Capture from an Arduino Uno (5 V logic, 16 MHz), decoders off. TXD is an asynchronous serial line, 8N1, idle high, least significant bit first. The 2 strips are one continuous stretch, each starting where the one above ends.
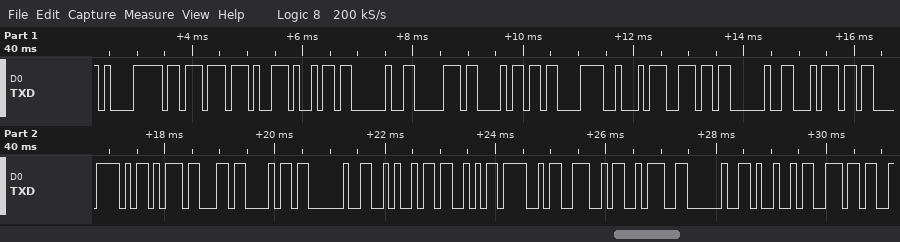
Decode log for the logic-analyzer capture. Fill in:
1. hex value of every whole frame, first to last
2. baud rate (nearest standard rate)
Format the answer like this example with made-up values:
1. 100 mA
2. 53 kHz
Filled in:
1. 0xE1 0xBB 0x97 0x69 0x20 0x70 0x68 0xC3 0xA2 0x6E 0x20 0x74 0xC3 0xAD 0x63 0x68 0x20 0x4A 0x53 0x4F 0x4E 0x3A 0x20 0x49 0x6E
2. 9600 baud
